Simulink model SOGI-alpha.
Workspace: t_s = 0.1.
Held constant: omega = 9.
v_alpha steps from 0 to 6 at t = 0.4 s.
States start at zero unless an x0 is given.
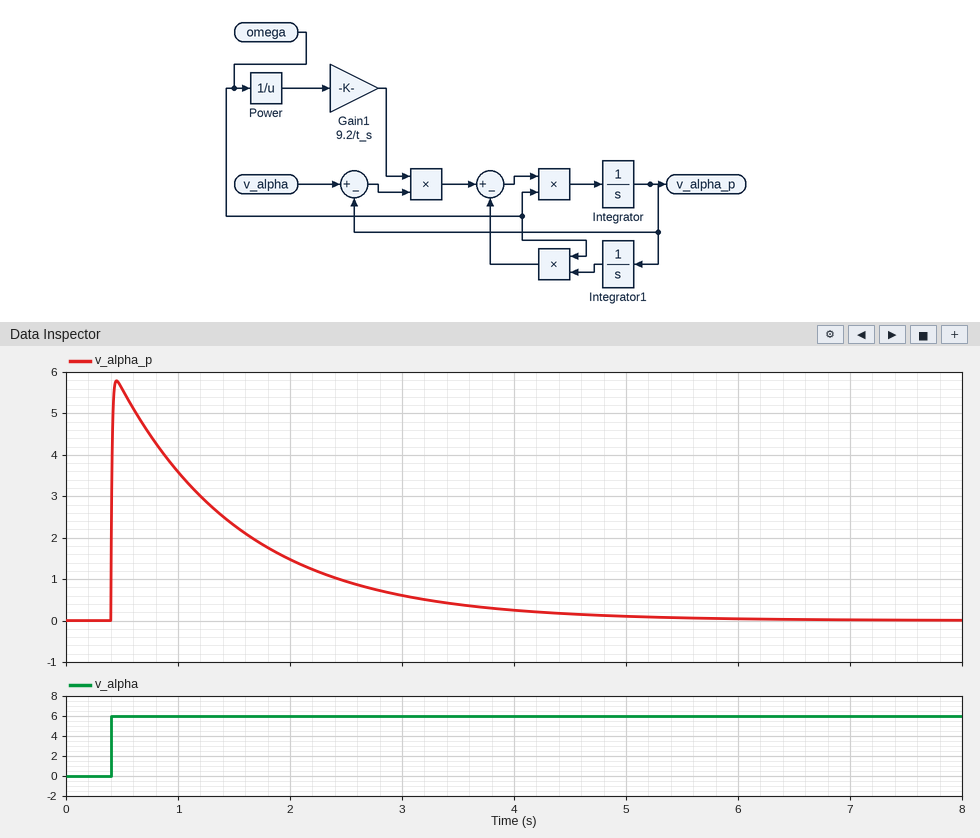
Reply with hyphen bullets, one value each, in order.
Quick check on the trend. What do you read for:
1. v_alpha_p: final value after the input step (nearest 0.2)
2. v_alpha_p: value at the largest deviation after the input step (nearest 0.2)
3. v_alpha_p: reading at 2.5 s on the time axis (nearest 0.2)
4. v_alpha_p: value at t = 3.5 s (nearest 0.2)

- 0.0
- 5.8
- 1.0
- 0.4
